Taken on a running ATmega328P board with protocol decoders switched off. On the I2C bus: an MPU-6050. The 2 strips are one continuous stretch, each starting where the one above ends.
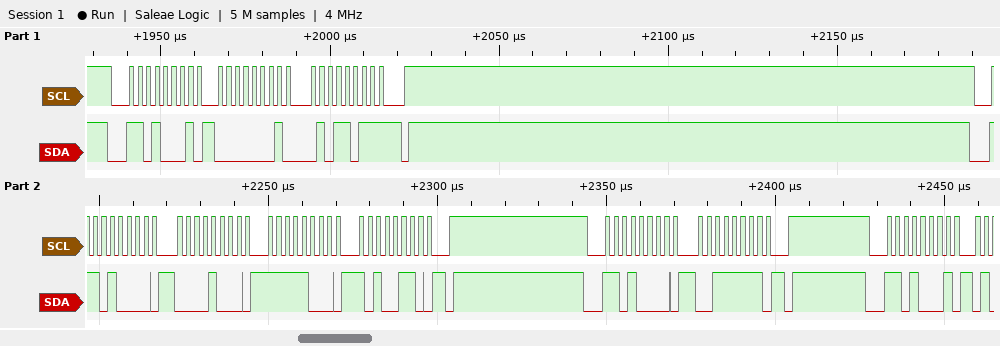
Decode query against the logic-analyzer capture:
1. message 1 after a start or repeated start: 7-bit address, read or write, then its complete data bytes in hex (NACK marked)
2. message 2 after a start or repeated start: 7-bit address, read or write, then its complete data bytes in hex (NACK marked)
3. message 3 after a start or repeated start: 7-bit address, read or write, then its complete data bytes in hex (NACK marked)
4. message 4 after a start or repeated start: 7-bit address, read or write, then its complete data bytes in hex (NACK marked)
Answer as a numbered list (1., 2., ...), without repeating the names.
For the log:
1. 0x68 read: 01 5B NACK
2. 0x68 write: 08 F8 A6
3. 0x68 write: 3F
4. 0x68 read
